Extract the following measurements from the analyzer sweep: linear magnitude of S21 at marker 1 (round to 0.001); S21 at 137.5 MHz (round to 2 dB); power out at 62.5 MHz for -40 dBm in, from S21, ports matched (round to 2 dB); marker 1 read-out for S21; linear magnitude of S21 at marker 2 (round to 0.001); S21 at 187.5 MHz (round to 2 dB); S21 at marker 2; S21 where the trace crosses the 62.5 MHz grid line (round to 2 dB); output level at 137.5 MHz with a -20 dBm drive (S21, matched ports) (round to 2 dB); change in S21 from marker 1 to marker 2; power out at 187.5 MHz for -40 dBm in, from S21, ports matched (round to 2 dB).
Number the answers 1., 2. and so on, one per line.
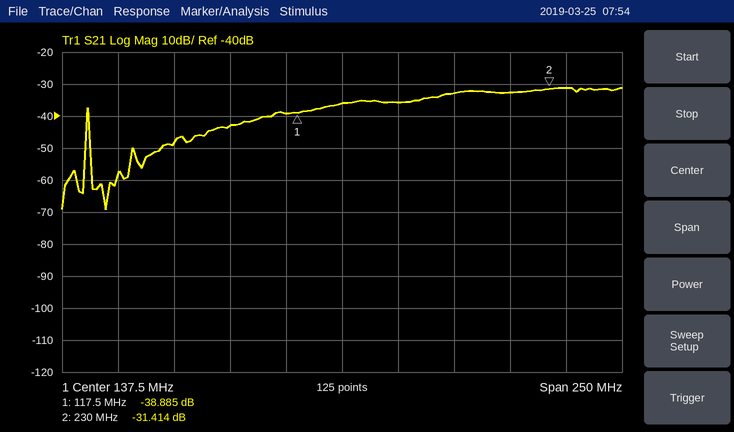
1. 0.011
2. -36 dB
3. -88 dBm
4. -38.885 dB
5. 0.027
6. -32 dB
7. -31.414 dB
8. -48 dB
9. -56 dBm
10. 7.471 dB
11. -72 dBm
